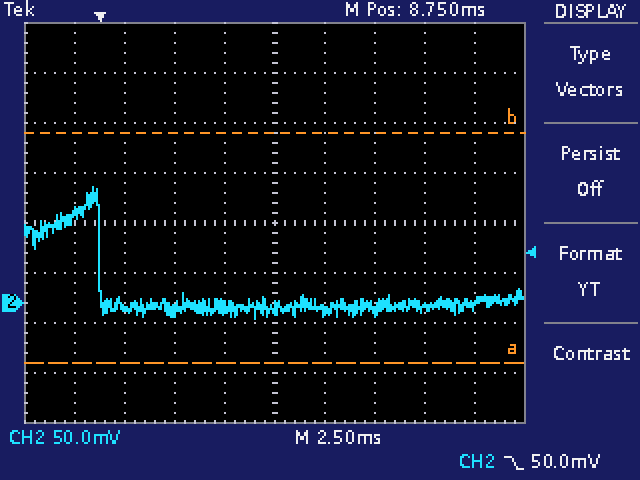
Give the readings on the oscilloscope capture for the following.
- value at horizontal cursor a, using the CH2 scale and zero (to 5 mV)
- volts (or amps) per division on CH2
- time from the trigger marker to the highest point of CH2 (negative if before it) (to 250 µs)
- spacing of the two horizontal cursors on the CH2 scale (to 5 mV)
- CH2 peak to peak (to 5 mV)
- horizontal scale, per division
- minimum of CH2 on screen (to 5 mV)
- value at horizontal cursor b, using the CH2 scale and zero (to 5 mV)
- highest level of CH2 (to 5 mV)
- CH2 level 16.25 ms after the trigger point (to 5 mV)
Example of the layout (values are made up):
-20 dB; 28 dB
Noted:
-60 mV; 50 mV; -250 µs; 230 mV; 130 mV; 2.5 ms; -15 mV; 170 mV; 115 mV; -5 mV
